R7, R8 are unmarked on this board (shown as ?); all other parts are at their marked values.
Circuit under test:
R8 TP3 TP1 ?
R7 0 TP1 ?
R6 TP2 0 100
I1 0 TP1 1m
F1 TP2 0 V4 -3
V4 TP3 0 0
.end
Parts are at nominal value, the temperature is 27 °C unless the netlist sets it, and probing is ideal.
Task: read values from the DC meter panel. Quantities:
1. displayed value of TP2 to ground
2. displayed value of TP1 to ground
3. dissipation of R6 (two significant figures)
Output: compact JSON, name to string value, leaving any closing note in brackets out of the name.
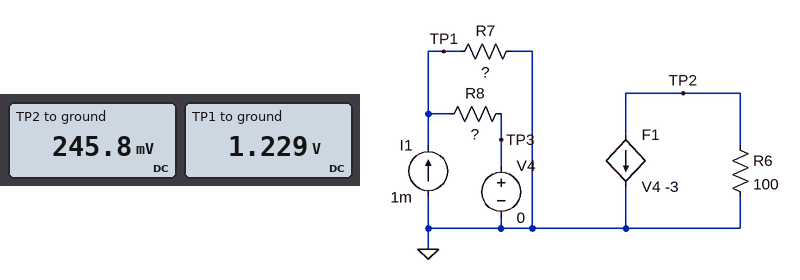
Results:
{"displayed value of TP2 to ground": "245.8 mV", "displayed value of TP1 to ground": "1.229 V", "dissipation of R6": "600 µW"}
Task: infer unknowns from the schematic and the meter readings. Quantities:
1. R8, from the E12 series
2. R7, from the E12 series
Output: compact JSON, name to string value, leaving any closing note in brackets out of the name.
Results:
{"R8, from the E12 series": "1.5 kΩ", "R7, from the E12 series": "6.8 kΩ"}
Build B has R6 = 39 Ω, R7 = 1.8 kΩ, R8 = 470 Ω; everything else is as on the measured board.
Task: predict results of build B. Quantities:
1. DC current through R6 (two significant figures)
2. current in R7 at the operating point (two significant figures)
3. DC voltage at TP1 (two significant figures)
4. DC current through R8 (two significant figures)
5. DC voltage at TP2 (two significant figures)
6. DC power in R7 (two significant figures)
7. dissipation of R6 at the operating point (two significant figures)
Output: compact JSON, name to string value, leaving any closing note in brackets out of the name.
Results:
{"DC current through R6": "2.4 mA", "current in R7 at the operating point": "210 µA", "DC voltage at TP1": "370 mV", "DC current through R8": "790 µA", "DC voltage at TP2": "93 mV", "DC power in R7": "77 µW", "dissipation of R6 at the operating point": "220 µW"}
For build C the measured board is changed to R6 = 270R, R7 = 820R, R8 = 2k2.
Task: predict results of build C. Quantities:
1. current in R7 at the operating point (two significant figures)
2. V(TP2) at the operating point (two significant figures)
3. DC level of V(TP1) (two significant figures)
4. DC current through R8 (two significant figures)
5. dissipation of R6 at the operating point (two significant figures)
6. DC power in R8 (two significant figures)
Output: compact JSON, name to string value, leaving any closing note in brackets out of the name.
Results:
{"current in R7 at the operating point": "730 µA", "V(TP2) at the operating point": "220 mV", "DC level of V(TP1)": "600 mV", "DC current through R8": "270 µA", "dissipation of R6 at the operating point": "180 µW", "DC power in R8": "160 µW"}
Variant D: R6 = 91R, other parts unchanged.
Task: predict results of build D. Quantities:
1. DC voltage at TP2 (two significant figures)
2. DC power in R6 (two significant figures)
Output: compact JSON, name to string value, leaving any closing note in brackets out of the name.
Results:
{"DC voltage at TP2": "220 mV", "DC power in R6": "550 µW"}
